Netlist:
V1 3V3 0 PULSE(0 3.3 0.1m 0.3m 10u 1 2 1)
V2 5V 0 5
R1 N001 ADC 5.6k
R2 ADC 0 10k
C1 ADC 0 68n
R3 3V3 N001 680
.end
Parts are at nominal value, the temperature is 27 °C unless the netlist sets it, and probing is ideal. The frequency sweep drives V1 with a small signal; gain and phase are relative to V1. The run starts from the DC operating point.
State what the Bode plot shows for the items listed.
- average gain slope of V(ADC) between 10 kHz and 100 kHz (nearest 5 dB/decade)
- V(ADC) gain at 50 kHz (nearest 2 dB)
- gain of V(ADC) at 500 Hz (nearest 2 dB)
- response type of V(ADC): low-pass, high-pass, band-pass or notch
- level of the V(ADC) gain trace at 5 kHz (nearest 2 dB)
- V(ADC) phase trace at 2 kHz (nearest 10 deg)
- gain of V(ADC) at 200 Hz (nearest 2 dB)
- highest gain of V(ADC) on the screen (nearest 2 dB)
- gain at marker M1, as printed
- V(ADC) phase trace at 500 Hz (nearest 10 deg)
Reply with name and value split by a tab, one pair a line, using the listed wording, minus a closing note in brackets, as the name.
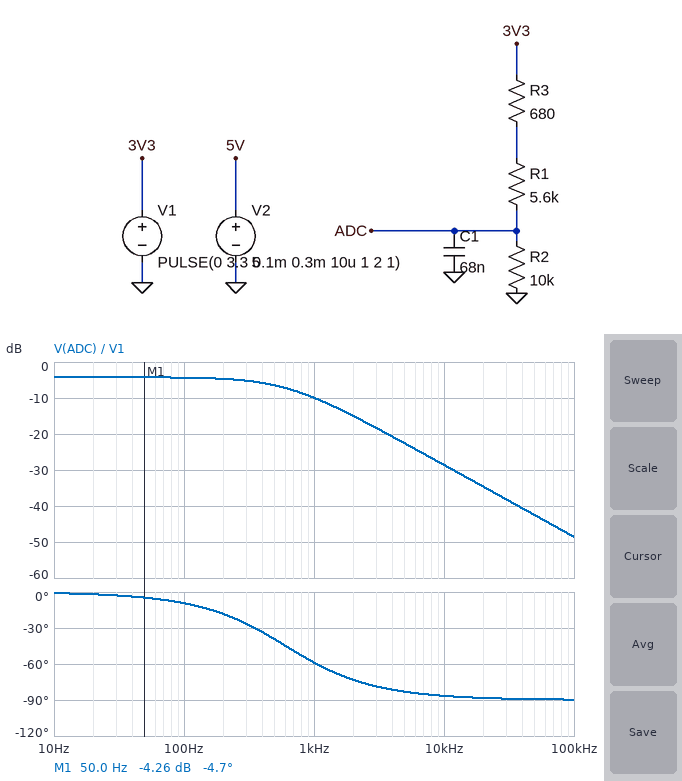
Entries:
average gain slope of V(ADC) between 10 kHz and 100 kHz	-20 dB/decade
V(ADC) gain at 50 kHz	-42 dB
gain of V(ADC) at 500 Hz	-6 dB
response type of V(ADC): low-pass, high-pass, band-pass or notch	low-pass
level of the V(ADC) gain trace at 5 kHz	-22 dB
V(ADC) phase trace at 2 kHz	-70 deg
gain of V(ADC) at 200 Hz	-4 dB
highest gain of V(ADC) on the screen	-4 dB
gain at marker M1, as printed	-4.26 dB
V(ADC) phase trace at 500 Hz	-40 deg
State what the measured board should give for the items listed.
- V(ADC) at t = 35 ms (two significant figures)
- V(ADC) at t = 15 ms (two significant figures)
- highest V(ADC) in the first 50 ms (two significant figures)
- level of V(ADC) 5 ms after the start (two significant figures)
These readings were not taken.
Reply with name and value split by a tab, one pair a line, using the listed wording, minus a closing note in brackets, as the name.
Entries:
V(ADC) at t = 35 ms	2.0 V
V(ADC) at t = 15 ms	2.0 V
highest V(ADC) in the first 50 ms	2.0 V
level of V(ADC) 5 ms after the start	2.0 V
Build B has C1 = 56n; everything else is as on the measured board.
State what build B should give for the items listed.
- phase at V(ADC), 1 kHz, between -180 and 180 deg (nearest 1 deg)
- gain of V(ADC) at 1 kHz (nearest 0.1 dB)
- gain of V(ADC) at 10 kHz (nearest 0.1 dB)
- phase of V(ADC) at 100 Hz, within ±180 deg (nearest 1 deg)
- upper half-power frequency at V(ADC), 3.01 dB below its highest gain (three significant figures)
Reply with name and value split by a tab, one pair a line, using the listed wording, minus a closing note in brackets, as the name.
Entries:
phase at V(ADC), 1 kHz, between -180 and 180 deg	-54 deg
gain of V(ADC) at 1 kHz	-8.8 dB
gain of V(ADC) at 10 kHz	-26.9 dB
phase of V(ADC) at 100 Hz, within ±180 deg	-8 deg
upper half-power frequency at V(ADC), 3.01 dB below its highest gain	737 Hz
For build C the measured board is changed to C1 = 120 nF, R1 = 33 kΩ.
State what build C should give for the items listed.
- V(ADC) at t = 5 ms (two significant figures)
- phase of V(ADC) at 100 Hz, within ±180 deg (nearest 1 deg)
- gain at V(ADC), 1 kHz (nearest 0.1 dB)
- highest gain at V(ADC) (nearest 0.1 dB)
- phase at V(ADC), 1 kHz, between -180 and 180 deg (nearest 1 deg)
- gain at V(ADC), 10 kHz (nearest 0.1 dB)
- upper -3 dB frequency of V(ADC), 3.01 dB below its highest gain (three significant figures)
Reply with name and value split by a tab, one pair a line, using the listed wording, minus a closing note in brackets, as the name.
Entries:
V(ADC) at t = 5 ms	750 mV
phase of V(ADC) at 100 Hz, within ±180 deg	-30 deg
gain at V(ADC), 1 kHz	-28.2 dB
highest gain at V(ADC)	-12.8 dB
phase at V(ADC), 1 kHz, between -180 and 180 deg	-80 deg
gain at V(ADC), 10 kHz	-48.1 dB
upper -3 dB frequency of V(ADC), 3.01 dB below its highest gain	172 Hz
